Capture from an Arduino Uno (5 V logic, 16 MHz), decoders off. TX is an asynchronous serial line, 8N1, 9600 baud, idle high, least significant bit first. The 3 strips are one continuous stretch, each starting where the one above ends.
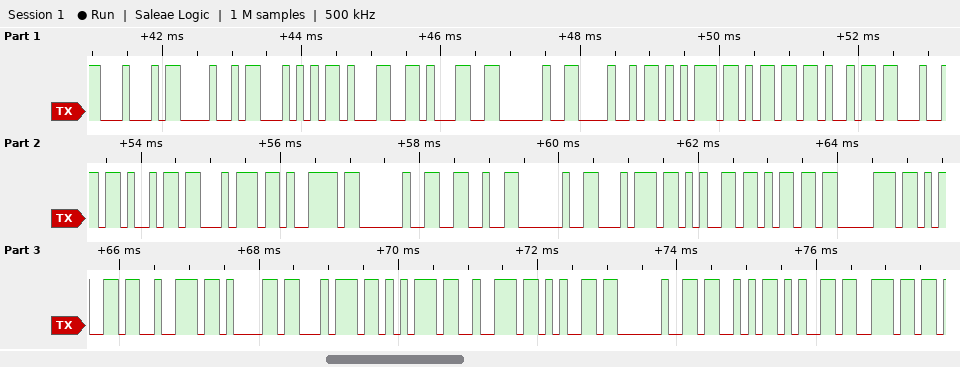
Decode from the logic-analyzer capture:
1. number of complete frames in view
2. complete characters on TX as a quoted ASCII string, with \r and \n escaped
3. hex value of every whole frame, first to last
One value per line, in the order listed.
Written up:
32
"DHT11 Humidity & temperature Sen"
44 48 54 31 31 20 48 75 6D 69 64 69 74 79 20 26 20 74 65 6D 70 65 72 61 74 75 72 65 20 53 65 6E
